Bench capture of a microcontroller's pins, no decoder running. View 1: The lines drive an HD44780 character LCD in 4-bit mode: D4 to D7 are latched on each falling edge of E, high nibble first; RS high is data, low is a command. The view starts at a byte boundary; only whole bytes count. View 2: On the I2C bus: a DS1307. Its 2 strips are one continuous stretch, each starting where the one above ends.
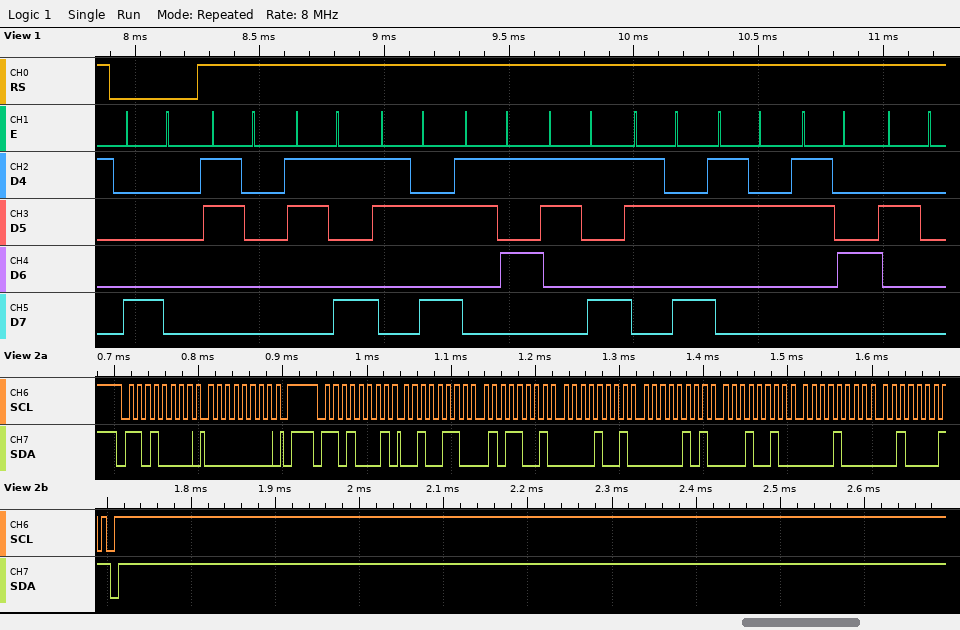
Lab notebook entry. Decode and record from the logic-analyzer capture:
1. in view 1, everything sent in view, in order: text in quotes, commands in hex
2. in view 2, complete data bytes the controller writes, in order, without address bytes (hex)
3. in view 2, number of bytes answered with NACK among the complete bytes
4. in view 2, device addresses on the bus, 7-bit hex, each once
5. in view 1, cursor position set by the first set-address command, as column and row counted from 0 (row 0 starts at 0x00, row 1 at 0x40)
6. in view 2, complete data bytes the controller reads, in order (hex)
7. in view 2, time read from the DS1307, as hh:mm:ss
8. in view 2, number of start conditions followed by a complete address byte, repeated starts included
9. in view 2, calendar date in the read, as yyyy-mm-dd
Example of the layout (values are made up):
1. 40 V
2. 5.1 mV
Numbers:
1. 0x80 "09:59:24 "
2. 00
3. 1
4. 0x68
5. column 0, row 0
6. 26 59 09 05 12 08 21
7. 09:59:26
8. 2
9. 2021-08-12
